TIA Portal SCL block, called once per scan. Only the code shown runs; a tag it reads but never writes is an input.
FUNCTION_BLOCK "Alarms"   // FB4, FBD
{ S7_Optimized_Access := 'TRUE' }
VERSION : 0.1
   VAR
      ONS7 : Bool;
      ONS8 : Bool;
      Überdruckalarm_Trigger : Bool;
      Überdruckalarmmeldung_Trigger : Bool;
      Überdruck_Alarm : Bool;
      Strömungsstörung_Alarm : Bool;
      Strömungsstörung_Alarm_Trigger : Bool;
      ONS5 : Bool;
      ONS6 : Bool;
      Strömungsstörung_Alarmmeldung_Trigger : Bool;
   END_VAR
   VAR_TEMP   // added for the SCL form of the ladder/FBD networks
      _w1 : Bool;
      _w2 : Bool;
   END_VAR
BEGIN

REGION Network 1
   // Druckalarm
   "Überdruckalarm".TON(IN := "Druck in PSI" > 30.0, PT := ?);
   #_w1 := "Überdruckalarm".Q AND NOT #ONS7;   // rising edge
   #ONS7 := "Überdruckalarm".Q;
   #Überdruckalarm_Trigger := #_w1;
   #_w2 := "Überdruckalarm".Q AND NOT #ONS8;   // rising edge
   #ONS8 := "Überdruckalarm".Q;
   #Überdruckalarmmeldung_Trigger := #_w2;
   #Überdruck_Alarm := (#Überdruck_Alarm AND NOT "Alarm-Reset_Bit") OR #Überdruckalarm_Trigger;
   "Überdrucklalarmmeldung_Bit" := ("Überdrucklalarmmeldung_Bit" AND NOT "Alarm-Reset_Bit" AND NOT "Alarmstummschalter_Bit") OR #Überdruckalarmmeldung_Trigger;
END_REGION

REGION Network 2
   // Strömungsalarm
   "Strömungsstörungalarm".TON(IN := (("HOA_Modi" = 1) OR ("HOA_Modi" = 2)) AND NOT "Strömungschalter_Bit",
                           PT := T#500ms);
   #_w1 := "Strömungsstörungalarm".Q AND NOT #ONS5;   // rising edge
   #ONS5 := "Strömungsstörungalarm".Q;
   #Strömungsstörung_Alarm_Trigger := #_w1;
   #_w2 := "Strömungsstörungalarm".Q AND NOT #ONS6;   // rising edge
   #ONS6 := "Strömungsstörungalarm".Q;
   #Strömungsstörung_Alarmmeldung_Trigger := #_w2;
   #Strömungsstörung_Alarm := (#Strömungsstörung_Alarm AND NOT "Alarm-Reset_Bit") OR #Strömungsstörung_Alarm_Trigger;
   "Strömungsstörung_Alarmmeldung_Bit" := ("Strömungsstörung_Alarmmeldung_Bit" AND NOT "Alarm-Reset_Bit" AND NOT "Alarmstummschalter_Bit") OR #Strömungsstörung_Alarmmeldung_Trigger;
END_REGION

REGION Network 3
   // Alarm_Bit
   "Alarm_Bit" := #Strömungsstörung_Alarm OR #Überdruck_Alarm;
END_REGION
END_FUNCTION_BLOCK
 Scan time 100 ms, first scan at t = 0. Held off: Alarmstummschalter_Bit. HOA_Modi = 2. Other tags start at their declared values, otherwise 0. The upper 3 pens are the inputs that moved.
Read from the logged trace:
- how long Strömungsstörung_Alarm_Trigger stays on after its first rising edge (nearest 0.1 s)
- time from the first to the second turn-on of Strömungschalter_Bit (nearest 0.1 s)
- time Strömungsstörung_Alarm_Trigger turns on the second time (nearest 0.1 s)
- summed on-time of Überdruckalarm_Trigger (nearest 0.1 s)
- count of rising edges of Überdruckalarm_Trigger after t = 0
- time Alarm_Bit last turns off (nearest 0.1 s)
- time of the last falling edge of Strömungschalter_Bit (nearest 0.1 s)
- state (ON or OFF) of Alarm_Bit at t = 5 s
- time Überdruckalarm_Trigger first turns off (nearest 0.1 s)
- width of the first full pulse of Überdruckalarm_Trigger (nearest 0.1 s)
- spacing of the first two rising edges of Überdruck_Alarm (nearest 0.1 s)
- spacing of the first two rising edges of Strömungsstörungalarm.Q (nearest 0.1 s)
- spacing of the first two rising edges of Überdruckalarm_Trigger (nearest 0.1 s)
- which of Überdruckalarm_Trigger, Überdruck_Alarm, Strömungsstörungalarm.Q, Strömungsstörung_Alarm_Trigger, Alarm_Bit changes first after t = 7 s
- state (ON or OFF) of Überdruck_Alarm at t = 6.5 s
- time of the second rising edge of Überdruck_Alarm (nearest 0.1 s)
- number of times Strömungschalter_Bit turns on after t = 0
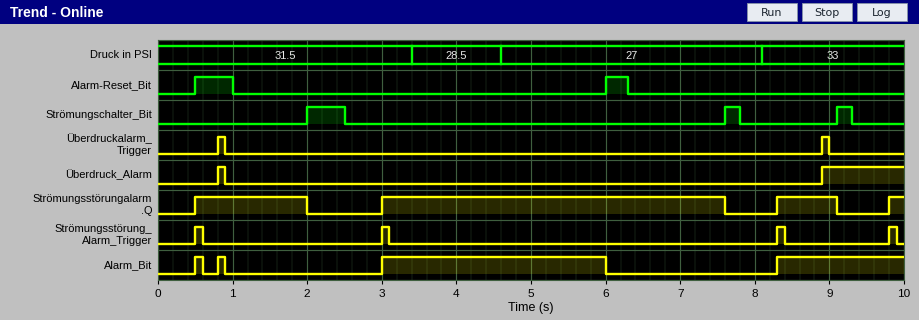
0.1 s
5.6 s
3.0 s
0.2 s
2
6.0 s
9.3 s
ON
0.9 s
0.1 s
8.1 s
2.5 s
8.1 s
Strömungsstörungalarm.Q
OFF
8.9 s
3
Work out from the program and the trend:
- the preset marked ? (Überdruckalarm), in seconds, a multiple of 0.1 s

0.8 s
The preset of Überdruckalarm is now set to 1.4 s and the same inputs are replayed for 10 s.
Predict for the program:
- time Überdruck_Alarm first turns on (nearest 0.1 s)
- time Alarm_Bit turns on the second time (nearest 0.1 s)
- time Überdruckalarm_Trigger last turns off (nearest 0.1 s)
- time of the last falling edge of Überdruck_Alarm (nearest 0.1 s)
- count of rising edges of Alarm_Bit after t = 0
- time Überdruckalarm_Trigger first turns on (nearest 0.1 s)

1.4 s
1.4 s
9.6 s
6.0 s
3
1.4 s
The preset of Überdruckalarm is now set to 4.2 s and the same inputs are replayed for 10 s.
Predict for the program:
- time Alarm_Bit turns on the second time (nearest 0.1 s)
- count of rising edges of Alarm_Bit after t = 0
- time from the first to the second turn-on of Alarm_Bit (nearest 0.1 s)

3.0 s
3
2.5 s
